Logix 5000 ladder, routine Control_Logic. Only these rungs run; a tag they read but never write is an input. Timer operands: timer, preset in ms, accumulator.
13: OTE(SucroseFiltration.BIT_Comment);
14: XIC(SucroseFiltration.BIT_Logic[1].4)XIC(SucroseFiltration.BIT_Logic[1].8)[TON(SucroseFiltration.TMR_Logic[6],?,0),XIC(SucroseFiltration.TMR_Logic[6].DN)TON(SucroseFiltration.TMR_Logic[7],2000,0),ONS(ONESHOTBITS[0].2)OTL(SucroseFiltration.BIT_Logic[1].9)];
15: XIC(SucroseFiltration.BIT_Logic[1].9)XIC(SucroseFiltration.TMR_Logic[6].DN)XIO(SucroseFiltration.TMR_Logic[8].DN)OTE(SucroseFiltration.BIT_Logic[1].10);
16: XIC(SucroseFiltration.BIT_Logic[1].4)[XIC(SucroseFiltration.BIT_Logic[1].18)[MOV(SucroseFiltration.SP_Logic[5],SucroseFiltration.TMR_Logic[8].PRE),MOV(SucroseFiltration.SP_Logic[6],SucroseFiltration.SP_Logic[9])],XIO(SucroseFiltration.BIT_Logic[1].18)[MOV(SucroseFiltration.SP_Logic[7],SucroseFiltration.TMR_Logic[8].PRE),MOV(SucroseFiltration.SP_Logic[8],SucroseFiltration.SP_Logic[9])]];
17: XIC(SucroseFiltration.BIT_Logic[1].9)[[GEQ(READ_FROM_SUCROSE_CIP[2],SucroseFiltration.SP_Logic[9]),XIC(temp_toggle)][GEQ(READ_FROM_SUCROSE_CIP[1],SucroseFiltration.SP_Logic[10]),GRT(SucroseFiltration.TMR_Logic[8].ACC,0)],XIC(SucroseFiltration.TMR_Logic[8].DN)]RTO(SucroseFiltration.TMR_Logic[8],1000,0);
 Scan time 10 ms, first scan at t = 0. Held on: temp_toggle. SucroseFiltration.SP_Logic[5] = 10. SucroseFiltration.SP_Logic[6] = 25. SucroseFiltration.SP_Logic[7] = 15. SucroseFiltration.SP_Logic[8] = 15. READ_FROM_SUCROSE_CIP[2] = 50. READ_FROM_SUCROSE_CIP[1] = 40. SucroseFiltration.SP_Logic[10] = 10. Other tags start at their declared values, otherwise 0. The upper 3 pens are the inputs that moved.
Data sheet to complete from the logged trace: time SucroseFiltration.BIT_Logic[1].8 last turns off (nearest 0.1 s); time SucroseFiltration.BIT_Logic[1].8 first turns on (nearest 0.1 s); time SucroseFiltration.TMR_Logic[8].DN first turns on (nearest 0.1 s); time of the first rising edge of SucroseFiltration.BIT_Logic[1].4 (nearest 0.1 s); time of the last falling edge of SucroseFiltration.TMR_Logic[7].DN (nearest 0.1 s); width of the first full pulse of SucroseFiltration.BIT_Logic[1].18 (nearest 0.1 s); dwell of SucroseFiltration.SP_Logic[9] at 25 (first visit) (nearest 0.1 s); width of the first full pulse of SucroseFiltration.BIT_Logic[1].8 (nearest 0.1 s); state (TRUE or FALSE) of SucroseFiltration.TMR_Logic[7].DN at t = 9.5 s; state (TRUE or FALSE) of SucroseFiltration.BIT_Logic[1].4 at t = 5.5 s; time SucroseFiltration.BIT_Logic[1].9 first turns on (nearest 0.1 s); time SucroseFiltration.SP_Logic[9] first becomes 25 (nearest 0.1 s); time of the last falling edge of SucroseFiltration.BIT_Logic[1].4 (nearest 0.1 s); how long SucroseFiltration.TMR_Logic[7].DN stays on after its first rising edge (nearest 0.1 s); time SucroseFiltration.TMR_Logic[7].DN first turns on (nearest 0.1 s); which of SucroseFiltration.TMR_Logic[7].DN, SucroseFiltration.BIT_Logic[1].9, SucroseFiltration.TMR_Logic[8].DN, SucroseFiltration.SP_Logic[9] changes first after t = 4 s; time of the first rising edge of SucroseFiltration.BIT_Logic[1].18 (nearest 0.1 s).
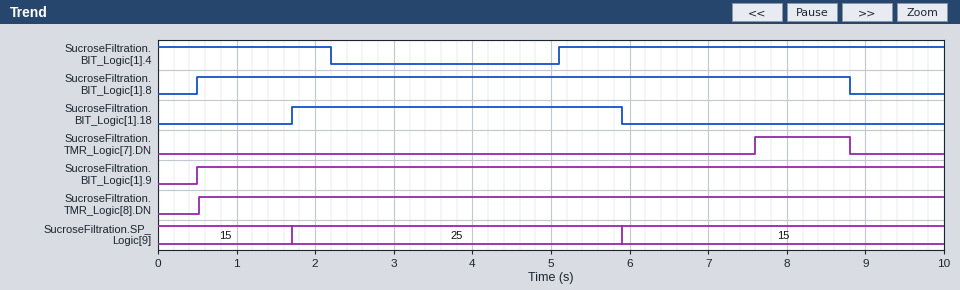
8.8 s
0.5 s
0.5 s
5.1 s
8.8 s
4.2 s
4.2 s
8.3 s
FALSE
TRUE
0.5 s
1.7 s
2.2 s
1.2 s
7.6 s
SucroseFiltration.SP_Logic[9]
1.7 s
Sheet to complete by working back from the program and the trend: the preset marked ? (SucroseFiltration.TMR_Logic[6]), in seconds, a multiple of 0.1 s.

0.5 s
